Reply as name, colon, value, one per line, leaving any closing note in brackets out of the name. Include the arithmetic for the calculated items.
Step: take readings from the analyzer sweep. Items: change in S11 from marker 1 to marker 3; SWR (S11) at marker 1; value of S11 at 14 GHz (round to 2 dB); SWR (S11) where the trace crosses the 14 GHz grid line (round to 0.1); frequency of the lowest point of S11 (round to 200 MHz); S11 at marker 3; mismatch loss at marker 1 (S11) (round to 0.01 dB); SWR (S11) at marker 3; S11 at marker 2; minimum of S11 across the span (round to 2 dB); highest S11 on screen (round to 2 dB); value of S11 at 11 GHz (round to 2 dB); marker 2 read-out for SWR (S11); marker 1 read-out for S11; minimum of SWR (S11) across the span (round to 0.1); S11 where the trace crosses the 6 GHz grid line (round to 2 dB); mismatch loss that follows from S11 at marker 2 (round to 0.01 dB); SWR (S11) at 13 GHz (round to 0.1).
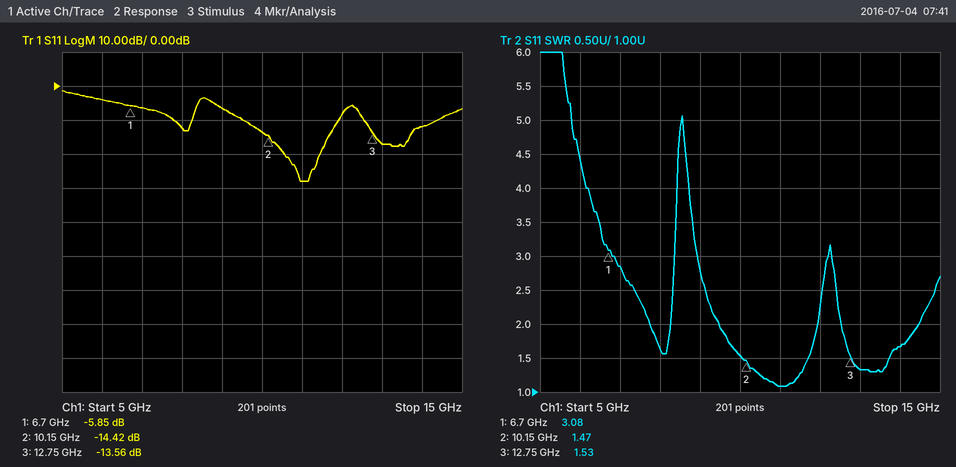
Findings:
change in S11 from marker 1 to marker 3: -13.56 − (-5.85) = -7.71 dB
SWR (S11) at marker 1: 3.08
value of S11 at 14 GHz: -12 dB
SWR (S11) where the trace crosses the 14 GHz grid line: 1.7
frequency of the lowest point of S11: 11.0 GHz
S11 at marker 3: -13.56 dB
mismatch loss at marker 1 (S11): −10 log10(1 − 10^(-5.85/10)) ≈ 1.31 dB
SWR (S11) at marker 3: 1.53
S11 at marker 2: -14.42 dB
minimum of S11 across the span: -28 dB
highest S11 on screen: -2 dB
value of S11 at 11 GHz: -28 dB
marker 2 read-out for SWR: 1.47
marker 1 read-out for S11: -5.85 dB
minimum of SWR (S11) across the span: 1.1
S11 where the trace crosses the 6 GHz grid line: -4 dB
mismatch loss that follows from S11 at marker 2: −10 log10(1 − 10^(-14.42/10)) ≈ 0.16 dB
SWR (S11) at 13 GHz: 1.3
